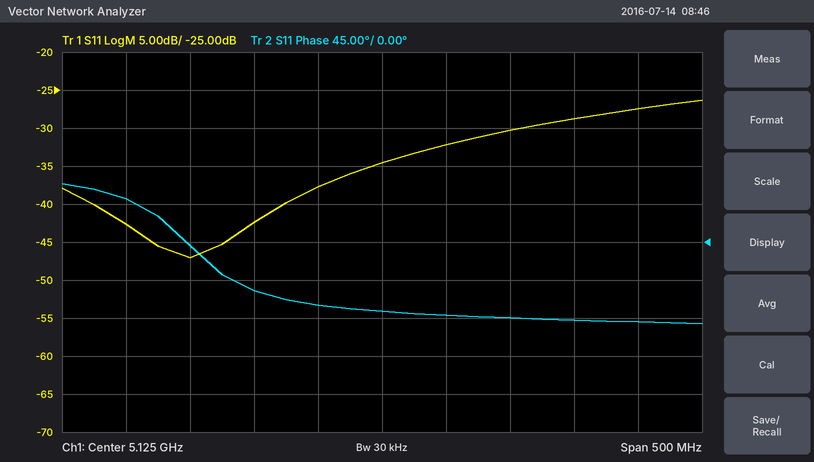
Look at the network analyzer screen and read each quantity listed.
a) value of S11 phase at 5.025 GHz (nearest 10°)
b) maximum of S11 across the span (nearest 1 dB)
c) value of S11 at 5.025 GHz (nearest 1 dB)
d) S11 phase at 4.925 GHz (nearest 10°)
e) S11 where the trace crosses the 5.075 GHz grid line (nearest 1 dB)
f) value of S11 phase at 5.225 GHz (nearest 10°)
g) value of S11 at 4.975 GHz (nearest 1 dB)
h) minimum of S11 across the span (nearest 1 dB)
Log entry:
-60°
-26 dB
-42 dB
50°
-38 dB
-90°
-47 dB
-47 dB
